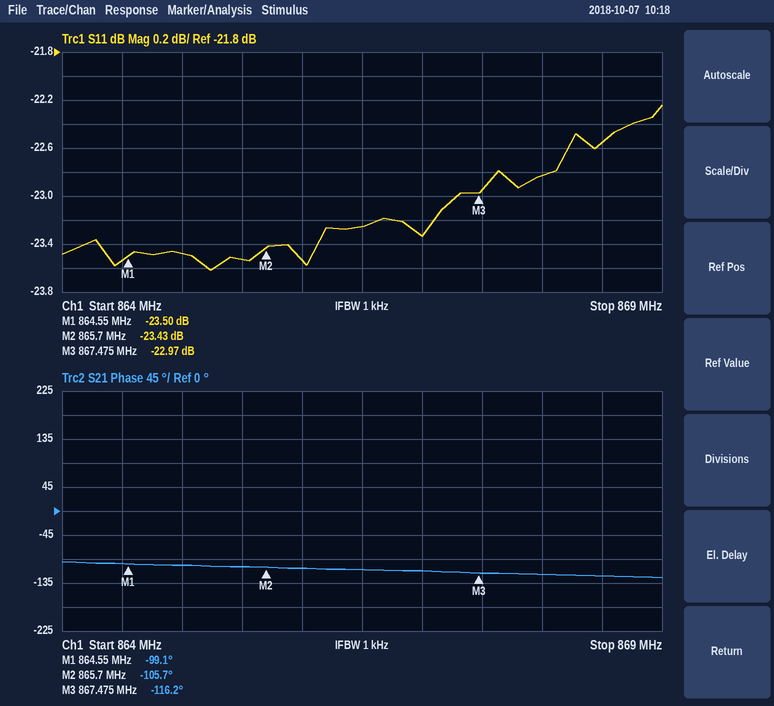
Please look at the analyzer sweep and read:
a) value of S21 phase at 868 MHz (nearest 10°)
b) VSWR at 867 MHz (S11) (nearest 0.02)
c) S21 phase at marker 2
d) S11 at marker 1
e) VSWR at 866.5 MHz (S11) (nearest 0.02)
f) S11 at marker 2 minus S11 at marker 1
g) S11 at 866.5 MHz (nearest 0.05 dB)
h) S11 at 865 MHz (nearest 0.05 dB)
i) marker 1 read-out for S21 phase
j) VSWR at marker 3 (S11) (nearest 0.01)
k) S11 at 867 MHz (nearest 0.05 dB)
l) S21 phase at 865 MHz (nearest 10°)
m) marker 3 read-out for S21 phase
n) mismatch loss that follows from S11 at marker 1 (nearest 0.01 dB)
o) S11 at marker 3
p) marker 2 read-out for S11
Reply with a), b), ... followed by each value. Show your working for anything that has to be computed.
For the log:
a) -120°
b) |Γ| = 10^(-23.35/20) = 0.0680; VSWR = (1 + 0.0680)/(1 − 0.0680) ≈ 1.15, so 1.14 to the nearest 0.02
c) -105.7°
d) -23.50 dB
e) |Γ| = 10^(-23.25/20) = 0.0688; VSWR = (1 + 0.0688)/(1 − 0.0688) ≈ 1.15, so 1.14 to the nearest 0.02
f) -23.43 − (-23.5) = 0.07 dB
g) -23.25 dB
h) -23.50 dB
i) -99.1°
j) (1 + 0.0710)/(1 − 0.0710) ≈ 1.15
k) -23.35 dB
l) -100°
m) -116.2°
n) −10 log10(1 − 10^(-23.5/10)) ≈ 0.02 dB
o) -22.97 dB
p) -23.43 dB
